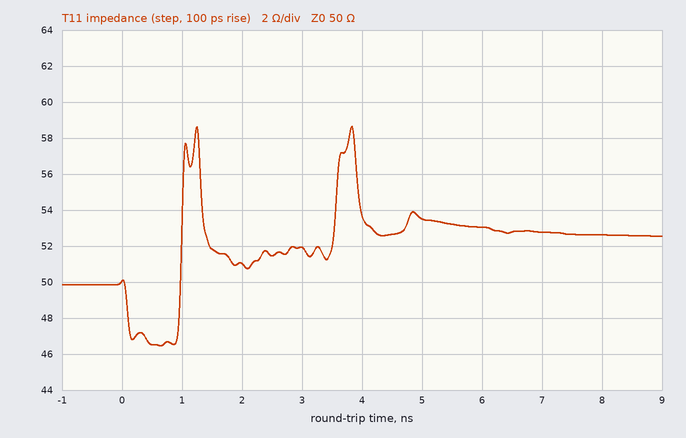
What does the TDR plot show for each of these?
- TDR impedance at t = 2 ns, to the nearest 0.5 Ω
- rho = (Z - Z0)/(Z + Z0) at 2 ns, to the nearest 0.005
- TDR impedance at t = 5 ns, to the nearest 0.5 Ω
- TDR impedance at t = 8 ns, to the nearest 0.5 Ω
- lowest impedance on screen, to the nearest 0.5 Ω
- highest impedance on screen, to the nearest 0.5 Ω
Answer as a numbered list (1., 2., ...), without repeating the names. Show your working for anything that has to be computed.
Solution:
1. 51.0 Ω
2. (51 − 50)/(51 + 50) ≈ +0.010
3. 53.5 Ω
4. 52.5 Ω
5. 46.5 Ω
6. 58.5 Ω
